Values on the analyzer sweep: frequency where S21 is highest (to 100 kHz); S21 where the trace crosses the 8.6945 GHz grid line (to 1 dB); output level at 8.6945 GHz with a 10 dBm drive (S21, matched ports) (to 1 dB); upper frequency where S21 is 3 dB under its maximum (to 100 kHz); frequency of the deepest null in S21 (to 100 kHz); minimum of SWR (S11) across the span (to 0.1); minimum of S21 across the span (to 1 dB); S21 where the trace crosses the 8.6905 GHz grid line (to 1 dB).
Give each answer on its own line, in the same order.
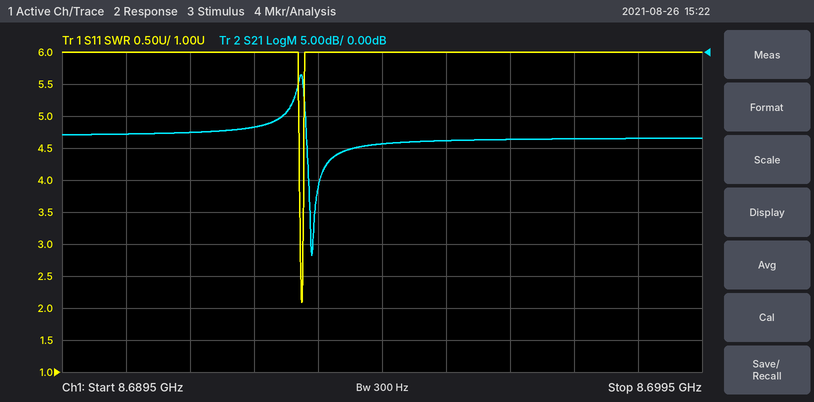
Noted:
8.6932 GHz
-14 dB
-4 dBm
8.6933 GHz
8.6934 GHz
2.1
-32 dB
-13 dB
